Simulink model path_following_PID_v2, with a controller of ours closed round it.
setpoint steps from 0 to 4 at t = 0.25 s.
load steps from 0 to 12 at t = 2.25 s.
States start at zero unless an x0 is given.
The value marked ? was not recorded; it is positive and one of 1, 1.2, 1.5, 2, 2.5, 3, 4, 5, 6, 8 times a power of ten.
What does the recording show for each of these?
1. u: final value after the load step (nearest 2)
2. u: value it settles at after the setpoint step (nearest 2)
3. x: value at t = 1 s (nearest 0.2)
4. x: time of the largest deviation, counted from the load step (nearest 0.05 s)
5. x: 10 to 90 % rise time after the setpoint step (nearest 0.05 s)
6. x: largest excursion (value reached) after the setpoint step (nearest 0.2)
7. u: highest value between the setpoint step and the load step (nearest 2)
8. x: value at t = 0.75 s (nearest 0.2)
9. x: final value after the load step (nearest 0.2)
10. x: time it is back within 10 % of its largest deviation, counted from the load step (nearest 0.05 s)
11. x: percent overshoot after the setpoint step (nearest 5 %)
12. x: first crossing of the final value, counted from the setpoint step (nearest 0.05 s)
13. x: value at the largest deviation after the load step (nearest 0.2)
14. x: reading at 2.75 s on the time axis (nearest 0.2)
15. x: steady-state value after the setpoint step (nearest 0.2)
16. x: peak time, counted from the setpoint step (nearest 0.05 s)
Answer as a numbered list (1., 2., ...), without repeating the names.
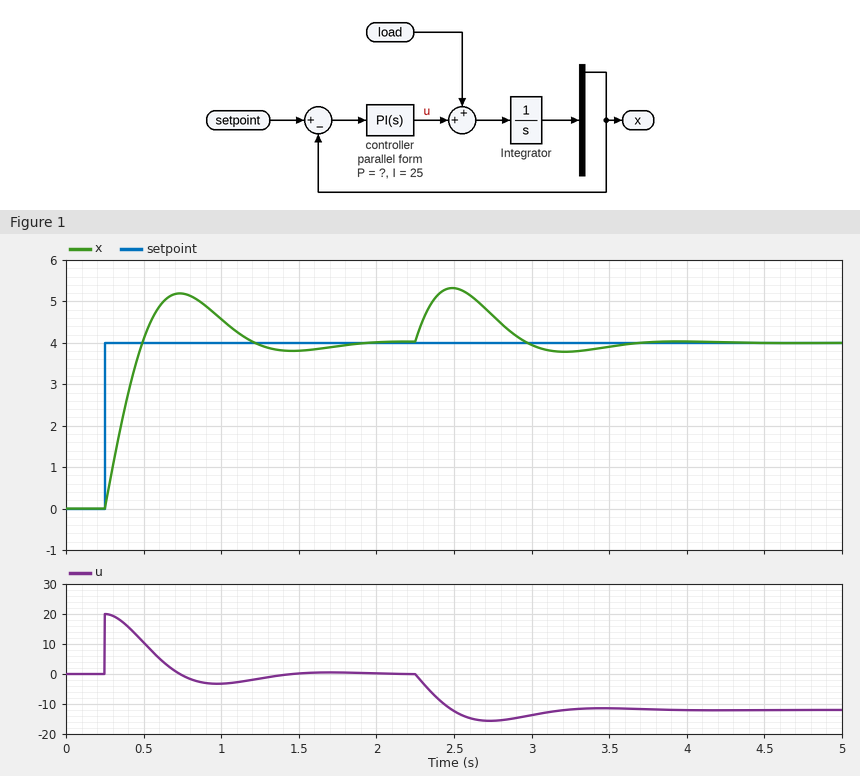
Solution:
1. -12
2. 0
3. 4.6
4. 0.25 s
5. 0.20 s
6. 5.2
7. 20
8. 5.2
9. 4.0
10. 1.20 s
11. 30 %
12. 0.25 s
13. 5.4
14. 4.6
15. 4.0
16. 0.50 s
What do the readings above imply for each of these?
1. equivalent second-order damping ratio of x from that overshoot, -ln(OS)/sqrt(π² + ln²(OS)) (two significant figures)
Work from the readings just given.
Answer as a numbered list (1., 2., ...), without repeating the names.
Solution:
1. 0.36
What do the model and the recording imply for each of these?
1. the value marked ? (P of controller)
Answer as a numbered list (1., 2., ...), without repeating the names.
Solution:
1. 5
